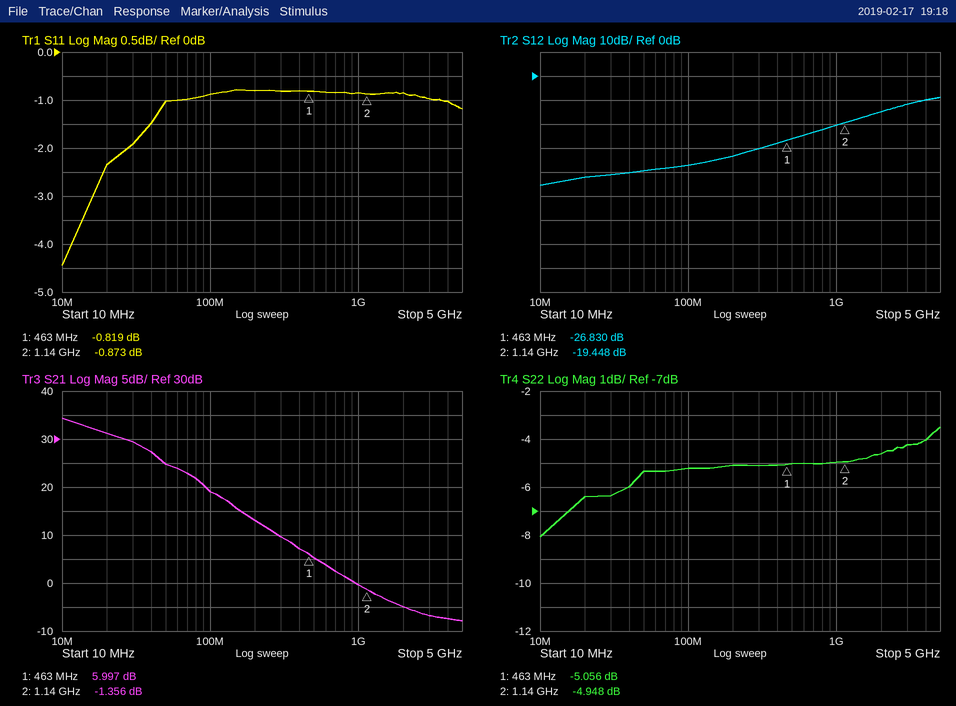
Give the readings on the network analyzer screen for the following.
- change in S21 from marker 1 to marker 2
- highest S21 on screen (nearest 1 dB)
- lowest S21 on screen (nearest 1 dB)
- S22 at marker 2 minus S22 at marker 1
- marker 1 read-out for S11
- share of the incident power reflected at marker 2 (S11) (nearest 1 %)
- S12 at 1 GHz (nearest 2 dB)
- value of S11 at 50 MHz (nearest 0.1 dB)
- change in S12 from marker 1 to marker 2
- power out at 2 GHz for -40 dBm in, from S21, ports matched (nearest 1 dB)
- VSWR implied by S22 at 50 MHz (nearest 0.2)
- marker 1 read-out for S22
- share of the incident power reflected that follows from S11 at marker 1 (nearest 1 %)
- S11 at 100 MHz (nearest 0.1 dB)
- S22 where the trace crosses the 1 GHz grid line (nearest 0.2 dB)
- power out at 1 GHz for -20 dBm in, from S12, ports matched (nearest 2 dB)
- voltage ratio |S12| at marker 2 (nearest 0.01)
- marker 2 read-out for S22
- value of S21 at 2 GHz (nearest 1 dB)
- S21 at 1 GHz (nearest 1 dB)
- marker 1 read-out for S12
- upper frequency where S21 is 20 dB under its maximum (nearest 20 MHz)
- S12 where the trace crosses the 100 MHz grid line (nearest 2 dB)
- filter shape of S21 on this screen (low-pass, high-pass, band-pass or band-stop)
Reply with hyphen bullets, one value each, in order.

- -7.353 dB
- 34 dB
- -8 dB
- 0.108 dB
- -0.819 dB
- 82 %
- -20 dB
- -1.0 dB
- 7.382 dB
- -45 dBm
- 3.4
- -5.056 dB
- 83 %
- -0.9 dB
- -5.0 dB
- -40 dBm
- 0.11
- -4.948 dB
- -5 dB
- 0 dB
- -26.830 dB
- 180 MHz
- -38 dB
- low-pass
